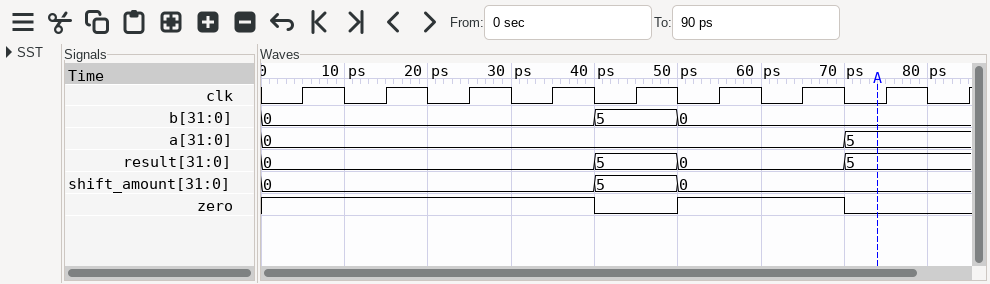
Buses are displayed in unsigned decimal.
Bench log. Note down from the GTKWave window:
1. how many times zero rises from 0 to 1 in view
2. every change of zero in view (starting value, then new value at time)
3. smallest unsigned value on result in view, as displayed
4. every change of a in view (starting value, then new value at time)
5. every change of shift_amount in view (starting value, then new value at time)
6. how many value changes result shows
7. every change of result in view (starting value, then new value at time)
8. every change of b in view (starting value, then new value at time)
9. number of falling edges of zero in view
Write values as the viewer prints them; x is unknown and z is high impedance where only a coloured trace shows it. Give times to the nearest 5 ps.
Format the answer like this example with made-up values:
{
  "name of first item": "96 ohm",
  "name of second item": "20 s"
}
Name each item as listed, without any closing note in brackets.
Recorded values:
{
  "how many times zero rises from 0 to 1 in view": "1",
  "every change of zero in view": "1, 0 at 40 ps, 1 at 50 ps, 0 at 70 ps",
  "smallest unsigned value on result in view, as displayed": "0",
  "every change of a in view": "0, 5 at 70 ps",
  "every change of shift_amount in view": "0, 5 at 40 ps, 0 at 50 ps",
  "how many value changes result shows": "3",
  "every change of result in view": "0, 5 at 40 ps, 0 at 50 ps, 5 at 70 ps",
  "every change of b in view": "0, 5 at 40 ps, 0 at 50 ps",
  "number of falling edges of zero in view": "2"
}
